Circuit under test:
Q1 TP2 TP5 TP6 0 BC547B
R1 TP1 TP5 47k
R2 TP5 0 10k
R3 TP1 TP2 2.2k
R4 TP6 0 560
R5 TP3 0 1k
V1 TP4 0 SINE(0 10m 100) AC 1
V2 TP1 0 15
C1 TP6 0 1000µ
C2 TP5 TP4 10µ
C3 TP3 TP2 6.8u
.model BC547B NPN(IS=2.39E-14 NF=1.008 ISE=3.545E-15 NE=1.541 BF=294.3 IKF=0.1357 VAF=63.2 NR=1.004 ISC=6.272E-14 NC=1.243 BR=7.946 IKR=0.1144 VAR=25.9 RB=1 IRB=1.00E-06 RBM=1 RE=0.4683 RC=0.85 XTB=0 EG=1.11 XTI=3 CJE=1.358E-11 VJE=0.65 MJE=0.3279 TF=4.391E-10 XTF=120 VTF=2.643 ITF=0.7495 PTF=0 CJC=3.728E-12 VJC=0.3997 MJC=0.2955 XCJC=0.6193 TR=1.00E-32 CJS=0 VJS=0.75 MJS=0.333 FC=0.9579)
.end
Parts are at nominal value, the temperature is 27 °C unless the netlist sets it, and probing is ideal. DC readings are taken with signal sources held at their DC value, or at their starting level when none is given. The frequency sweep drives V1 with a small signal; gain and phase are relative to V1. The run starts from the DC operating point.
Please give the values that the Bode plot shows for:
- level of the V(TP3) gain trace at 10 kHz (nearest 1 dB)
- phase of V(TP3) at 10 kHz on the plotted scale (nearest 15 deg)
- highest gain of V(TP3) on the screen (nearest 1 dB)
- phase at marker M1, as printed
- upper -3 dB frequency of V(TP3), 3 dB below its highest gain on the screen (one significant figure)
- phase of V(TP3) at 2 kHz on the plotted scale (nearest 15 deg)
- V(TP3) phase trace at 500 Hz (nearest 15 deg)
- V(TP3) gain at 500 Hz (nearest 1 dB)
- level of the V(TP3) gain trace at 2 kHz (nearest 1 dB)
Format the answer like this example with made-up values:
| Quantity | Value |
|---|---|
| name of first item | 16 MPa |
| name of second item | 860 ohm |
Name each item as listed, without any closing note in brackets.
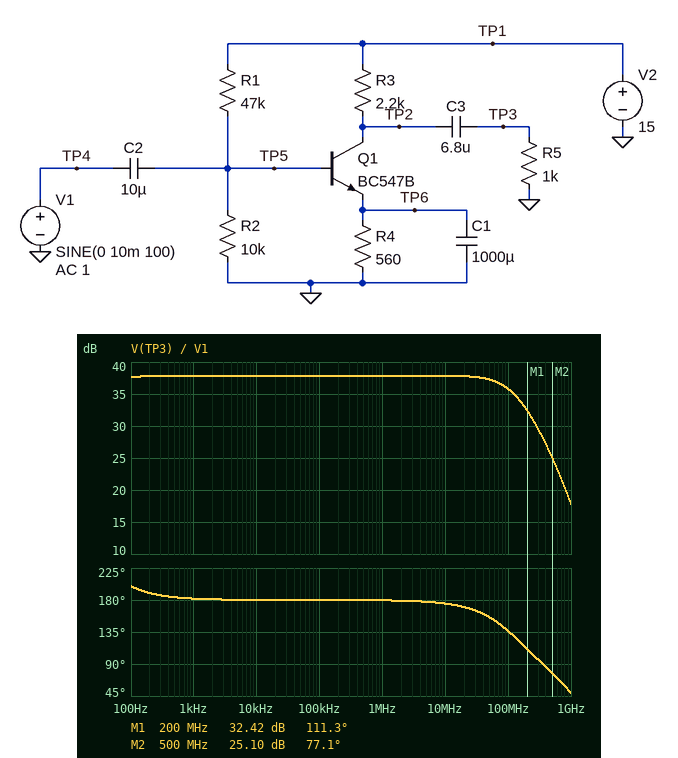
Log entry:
| Quantity | Value |
|---|---|
| level of the V(TP3) gain trace at 10 kHz | 38 dB |
| phase of V(TP3) at 10 kHz on the plotted scale | 180 deg |
| highest gain of V(TP3) on the screen | 38 dB |
| phase at marker M1, as printed | 111.3 deg |
| upper -3 dB frequency of V(TP3), 3 dB below its highest gain on the screen | 100 MHz |
| phase of V(TP3) at 2 kHz on the plotted scale | 180 deg |
| V(TP3) phase trace at 500 Hz | 180 deg |
| V(TP3) gain at 500 Hz | 38 dB |
| level of the V(TP3) gain trace at 2 kHz | 38 dB |
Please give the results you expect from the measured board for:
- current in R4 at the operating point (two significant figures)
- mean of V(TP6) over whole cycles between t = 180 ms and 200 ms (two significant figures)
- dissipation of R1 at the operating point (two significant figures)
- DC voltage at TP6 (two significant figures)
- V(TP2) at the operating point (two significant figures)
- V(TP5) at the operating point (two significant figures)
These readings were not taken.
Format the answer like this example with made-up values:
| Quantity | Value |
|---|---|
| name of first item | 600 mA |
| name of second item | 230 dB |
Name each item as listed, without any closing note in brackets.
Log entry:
| Quantity | Value |
|---|---|
| current in R4 at the operating point | 3.3 mA |
| mean of V(TP6) over whole cycles between t = 180 ms and 200 ms | 1.9 V |
| dissipation of R1 at the operating point | 3.3 mW |
| DC voltage at TP6 | 1.9 V |
| V(TP2) at the operating point | 7.7 V |
| V(TP5) at the operating point | 2.5 V |
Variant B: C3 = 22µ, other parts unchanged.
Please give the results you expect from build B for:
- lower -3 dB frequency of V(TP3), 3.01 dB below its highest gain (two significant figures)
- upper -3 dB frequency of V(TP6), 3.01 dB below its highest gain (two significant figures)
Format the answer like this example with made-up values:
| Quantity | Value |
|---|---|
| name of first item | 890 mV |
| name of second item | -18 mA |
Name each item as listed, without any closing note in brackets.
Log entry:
| Quantity | Value |
|---|---|
| lower -3 dB frequency of V(TP3), 3.01 dB below its highest gain | 26 Hz |
| upper -3 dB frequency of V(TP6), 3.01 dB below its highest gain | 28 Hz |
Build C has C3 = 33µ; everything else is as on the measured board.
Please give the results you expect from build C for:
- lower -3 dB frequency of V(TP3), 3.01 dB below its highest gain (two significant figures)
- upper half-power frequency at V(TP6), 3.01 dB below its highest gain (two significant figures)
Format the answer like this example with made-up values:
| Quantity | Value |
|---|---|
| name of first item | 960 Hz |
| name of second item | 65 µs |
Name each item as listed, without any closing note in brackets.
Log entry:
| Quantity | Value |
|---|---|
| lower -3 dB frequency of V(TP3), 3.01 dB below its highest gain | 26 Hz |
| upper half-power frequency at V(TP6), 3.01 dB below its highest gain | 28 Hz |
